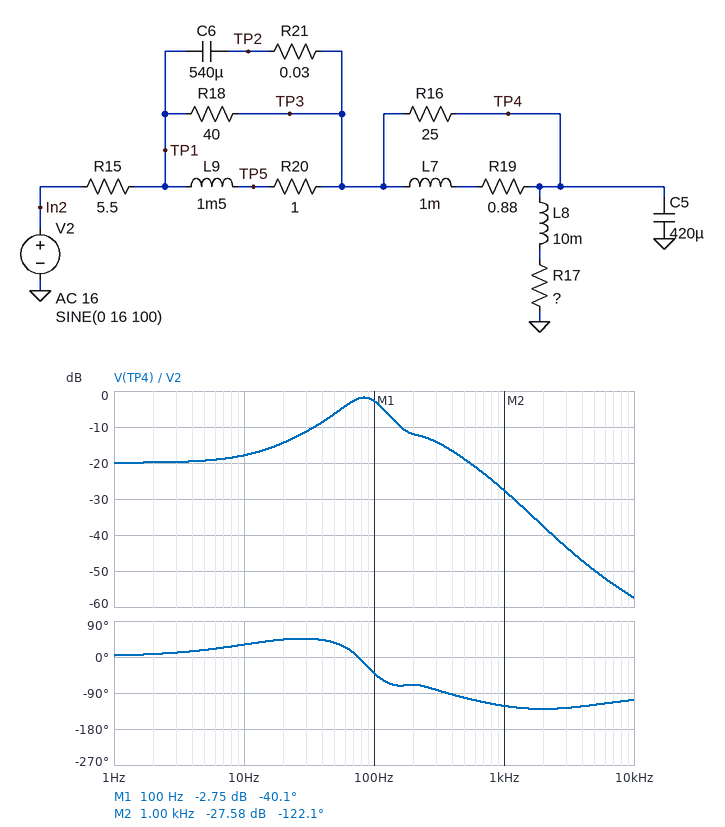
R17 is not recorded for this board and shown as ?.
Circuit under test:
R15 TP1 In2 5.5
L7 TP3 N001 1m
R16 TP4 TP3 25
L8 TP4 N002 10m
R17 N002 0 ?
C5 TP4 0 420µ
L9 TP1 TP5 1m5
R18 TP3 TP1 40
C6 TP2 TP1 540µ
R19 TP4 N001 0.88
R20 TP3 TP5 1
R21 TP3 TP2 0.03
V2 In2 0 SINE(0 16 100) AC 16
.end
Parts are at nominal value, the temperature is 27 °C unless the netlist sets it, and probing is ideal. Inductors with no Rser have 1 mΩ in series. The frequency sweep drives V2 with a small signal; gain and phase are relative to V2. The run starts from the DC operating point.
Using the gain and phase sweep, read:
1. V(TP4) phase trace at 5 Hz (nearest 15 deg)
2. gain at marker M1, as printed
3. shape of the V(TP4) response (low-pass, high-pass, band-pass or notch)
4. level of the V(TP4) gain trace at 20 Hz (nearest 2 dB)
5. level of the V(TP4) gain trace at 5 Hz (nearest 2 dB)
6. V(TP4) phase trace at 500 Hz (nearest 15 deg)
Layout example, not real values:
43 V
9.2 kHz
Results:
15 deg
-2.75 dB
band-pass
-14 dB
-20 dB
-105 deg
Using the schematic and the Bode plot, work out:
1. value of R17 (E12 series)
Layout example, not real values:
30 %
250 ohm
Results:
0.82 Ω
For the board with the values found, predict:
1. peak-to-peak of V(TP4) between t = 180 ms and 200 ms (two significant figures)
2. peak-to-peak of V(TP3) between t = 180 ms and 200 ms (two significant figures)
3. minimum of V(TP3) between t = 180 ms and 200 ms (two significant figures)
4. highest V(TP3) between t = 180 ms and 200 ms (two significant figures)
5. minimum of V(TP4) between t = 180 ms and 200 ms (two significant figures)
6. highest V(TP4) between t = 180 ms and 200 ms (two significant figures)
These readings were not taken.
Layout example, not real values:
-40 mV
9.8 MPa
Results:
23 V
22 V
-11 V
11 V
-12 V
12 V
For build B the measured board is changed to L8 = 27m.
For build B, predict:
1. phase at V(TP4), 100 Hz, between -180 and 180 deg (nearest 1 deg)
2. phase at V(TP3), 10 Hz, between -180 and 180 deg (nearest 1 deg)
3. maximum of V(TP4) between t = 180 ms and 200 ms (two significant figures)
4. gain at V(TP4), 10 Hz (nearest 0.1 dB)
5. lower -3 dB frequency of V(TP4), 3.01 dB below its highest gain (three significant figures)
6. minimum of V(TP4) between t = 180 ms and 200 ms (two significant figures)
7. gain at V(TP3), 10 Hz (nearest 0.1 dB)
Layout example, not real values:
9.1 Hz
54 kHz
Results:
-64 deg
33 deg
8.7 V
-12.6 dB
29.6 Hz
-8.7 V
-10.5 dB
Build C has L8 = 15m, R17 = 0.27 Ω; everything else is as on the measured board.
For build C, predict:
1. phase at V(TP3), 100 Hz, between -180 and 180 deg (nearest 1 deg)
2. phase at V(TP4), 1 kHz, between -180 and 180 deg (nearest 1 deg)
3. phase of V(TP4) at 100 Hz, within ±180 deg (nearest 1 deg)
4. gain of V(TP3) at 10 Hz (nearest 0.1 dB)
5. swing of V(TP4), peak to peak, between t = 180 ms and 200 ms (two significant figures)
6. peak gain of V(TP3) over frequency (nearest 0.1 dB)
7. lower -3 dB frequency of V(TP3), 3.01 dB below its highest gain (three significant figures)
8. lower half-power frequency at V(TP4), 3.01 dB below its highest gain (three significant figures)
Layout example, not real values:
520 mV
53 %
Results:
-47 deg
-122 deg
-56 deg
-14.0 dB
21 V
-0.4 dB
42.4 Hz
44.3 Hz
